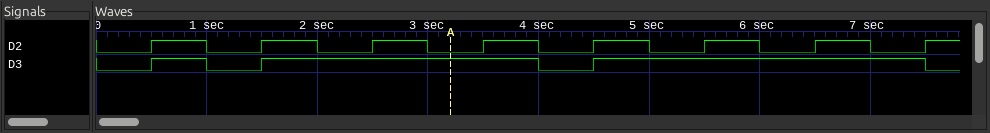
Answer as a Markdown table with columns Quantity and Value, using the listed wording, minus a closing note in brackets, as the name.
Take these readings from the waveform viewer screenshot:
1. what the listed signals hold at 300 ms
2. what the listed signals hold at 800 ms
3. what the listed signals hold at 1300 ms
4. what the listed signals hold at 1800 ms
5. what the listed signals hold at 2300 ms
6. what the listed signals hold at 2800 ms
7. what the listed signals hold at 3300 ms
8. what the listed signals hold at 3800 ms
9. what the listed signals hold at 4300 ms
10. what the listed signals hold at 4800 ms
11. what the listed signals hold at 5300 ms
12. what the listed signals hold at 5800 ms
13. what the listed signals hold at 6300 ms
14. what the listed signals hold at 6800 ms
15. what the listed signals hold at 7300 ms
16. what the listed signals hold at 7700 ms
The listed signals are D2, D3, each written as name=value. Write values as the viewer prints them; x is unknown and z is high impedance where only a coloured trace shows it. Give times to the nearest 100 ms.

| Quantity | Value |
|---|---|
| what the listed signals hold at 300 ms | D2=0, D3=0 |
| what the listed signals hold at 800 ms | D2=1, D3=1 |
| what the listed signals hold at 1300 ms | D2=0, D3=0 |
| what the listed signals hold at 1800 ms | D2=1, D3=1 |
| what the listed signals hold at 2300 ms | D2=0, D3=1 |
| what the listed signals hold at 2800 ms | D2=1, D3=1 |
| what the listed signals hold at 3300 ms | D2=0, D3=1 |
| what the listed signals hold at 3800 ms | D2=1, D3=1 |
| what the listed signals hold at 4300 ms | D2=0, D3=0 |
| what the listed signals hold at 4800 ms | D2=1, D3=1 |
| what the listed signals hold at 5300 ms | D2=0, D3=1 |
| what the listed signals hold at 5800 ms | D2=1, D3=1 |
| what the listed signals hold at 6300 ms | D2=0, D3=1 |
| what the listed signals hold at 6800 ms | D2=1, D3=1 |
| what the listed signals hold at 7300 ms | D2=0, D3=1 |
| what the listed signals hold at 7700 ms | D2=1, D3=0 |
